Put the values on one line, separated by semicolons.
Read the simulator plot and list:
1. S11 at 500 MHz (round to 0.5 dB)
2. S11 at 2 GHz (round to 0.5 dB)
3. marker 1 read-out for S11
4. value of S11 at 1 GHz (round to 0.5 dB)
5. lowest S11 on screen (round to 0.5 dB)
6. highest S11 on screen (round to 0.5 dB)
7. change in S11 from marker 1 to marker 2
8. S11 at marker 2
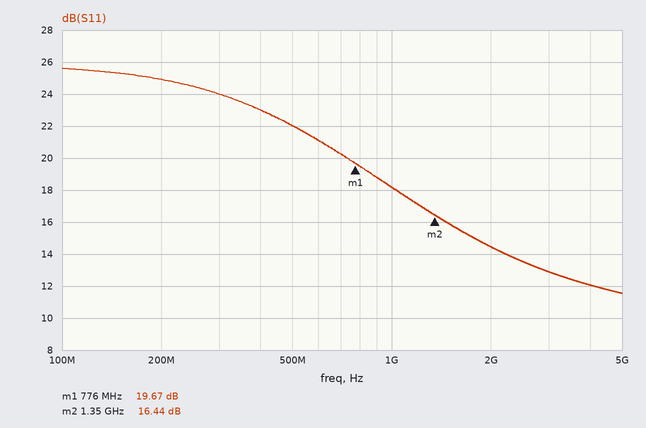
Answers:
22.0 dB; 14.5 dB; 19.67 dB; 18.0 dB; 11.5 dB; 25.5 dB; -3.23 dB; 16.44 dB
